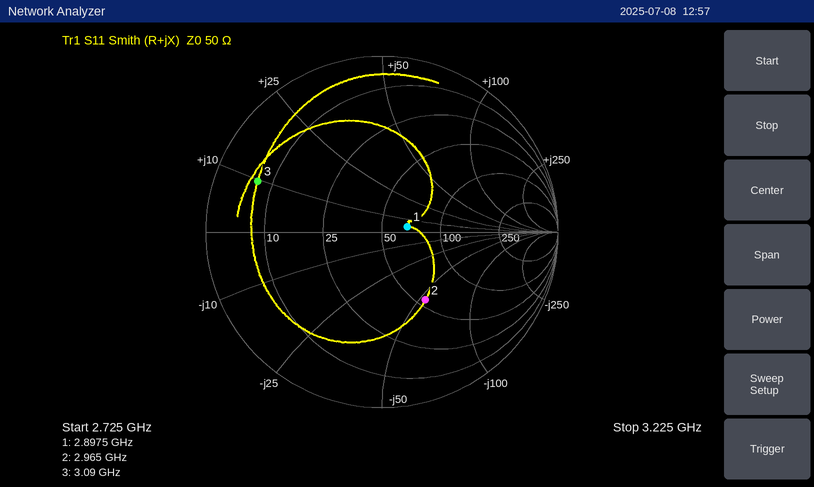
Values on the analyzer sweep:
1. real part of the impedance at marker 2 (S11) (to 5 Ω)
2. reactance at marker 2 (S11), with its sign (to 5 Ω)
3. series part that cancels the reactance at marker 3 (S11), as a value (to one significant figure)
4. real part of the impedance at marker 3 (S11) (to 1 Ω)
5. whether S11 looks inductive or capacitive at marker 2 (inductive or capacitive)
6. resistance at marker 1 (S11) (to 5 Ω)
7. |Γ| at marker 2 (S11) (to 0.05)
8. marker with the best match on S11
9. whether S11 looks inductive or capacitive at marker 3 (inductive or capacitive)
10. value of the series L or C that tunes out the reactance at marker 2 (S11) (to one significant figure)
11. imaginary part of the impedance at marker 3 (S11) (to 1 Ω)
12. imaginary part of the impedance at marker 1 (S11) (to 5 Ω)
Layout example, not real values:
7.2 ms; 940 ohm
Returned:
55 Ω; -55 Ω; 5 pF; 7 Ω; capacitive; 65 Ω; 0.45; marker 1; inductive; 3 nH; +10 Ω; +5 Ω
